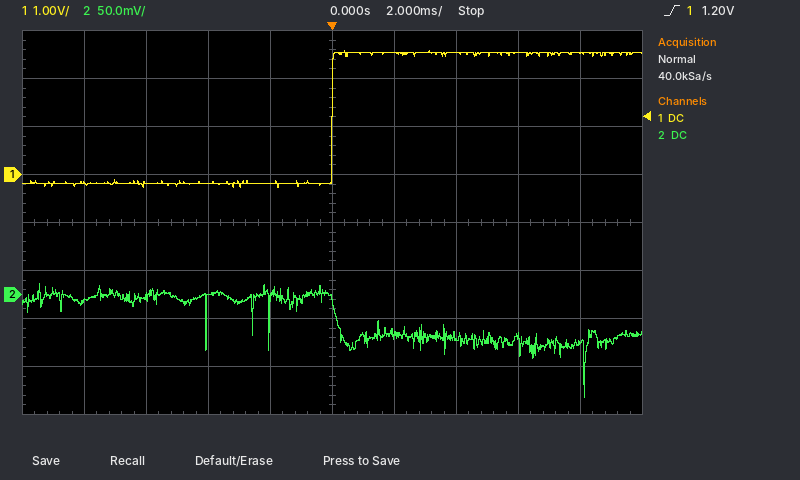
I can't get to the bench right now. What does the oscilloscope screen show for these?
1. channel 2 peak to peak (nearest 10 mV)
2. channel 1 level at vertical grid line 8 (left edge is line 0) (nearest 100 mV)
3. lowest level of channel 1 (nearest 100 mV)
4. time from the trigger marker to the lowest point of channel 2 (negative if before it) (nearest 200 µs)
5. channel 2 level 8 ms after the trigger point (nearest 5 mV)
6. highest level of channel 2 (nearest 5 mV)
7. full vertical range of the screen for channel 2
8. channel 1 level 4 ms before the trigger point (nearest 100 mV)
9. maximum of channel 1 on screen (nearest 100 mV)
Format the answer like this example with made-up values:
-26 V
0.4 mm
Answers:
120 mV
2.5 V
-300 mV
+8.2 ms
-50 mV
10 mV
400 mV
-200 mV
2.6 V
